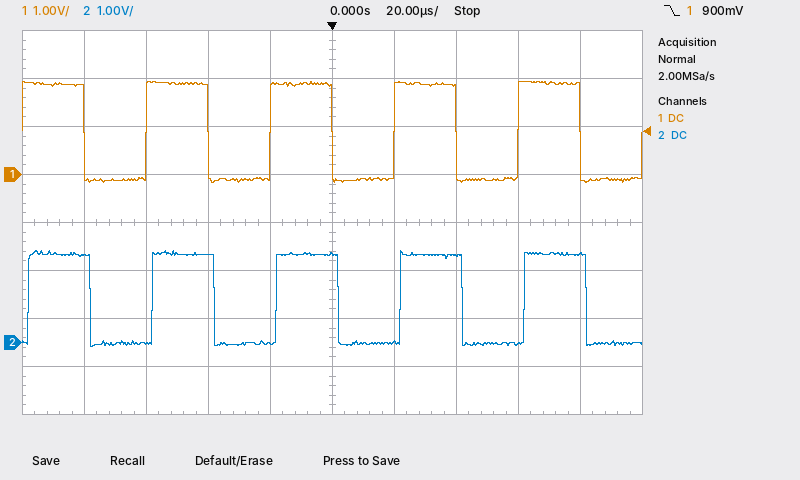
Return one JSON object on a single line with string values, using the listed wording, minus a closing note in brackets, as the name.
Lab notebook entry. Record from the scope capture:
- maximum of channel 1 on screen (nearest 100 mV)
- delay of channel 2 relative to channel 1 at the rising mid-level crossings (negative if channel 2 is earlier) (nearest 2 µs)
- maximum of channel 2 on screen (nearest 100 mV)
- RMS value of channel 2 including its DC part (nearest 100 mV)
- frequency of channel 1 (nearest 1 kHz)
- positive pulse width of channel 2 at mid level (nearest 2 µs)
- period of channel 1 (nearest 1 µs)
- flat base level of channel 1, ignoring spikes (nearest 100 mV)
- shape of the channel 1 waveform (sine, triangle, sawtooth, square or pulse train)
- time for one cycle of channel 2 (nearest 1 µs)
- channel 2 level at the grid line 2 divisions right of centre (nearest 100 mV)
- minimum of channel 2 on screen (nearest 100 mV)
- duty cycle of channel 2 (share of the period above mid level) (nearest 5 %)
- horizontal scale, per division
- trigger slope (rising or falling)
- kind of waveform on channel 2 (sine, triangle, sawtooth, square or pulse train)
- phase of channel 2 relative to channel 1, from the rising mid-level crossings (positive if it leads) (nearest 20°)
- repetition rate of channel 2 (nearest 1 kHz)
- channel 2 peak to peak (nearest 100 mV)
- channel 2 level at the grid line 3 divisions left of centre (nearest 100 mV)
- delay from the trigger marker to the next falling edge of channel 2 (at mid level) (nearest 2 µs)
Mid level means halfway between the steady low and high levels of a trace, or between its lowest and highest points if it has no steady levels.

{"maximum of channel 1 on screen": "1.9 V", "delay of channel 2 relative to channel 1 at the rising mid-level crossings (negative if channel 2 is earlier)": "+2 µs", "maximum of channel 2 on screen": "1.9 V", "RMS value of channel 2 including its DC part": "1.3 V", "frequency of channel 1": "25 kHz", "positive pulse width of channel 2 at mid level": "20 µs", "period of channel 1": "40 µs", "flat base level of channel 1, ignoring spikes": "-100 mV", "shape of the channel 1 waveform": "square", "time for one cycle of channel 2": "40 µs", "channel 2 level at the grid line 2 divisions right of centre": "1.8 V", "minimum of channel 2 on screen": "-100 mV", "duty cycle of channel 2 (share of the period above mid level)": "50 %", "horizontal scale, per division": "20 µs", "trigger slope": "falling", "kind of waveform on channel 2": "square", "phase of channel 2 relative to channel 1, from the rising mid-level crossings (positive if it leads)": "-20°", "repetition rate of channel 2": "25 kHz", "channel 2 peak to peak": "2.0 V", "channel 2 level at the grid line 3 divisions left of centre": "0.0 V", "delay from the trigger marker to the next falling edge of channel 2 (at mid level)": "2 µs"}
